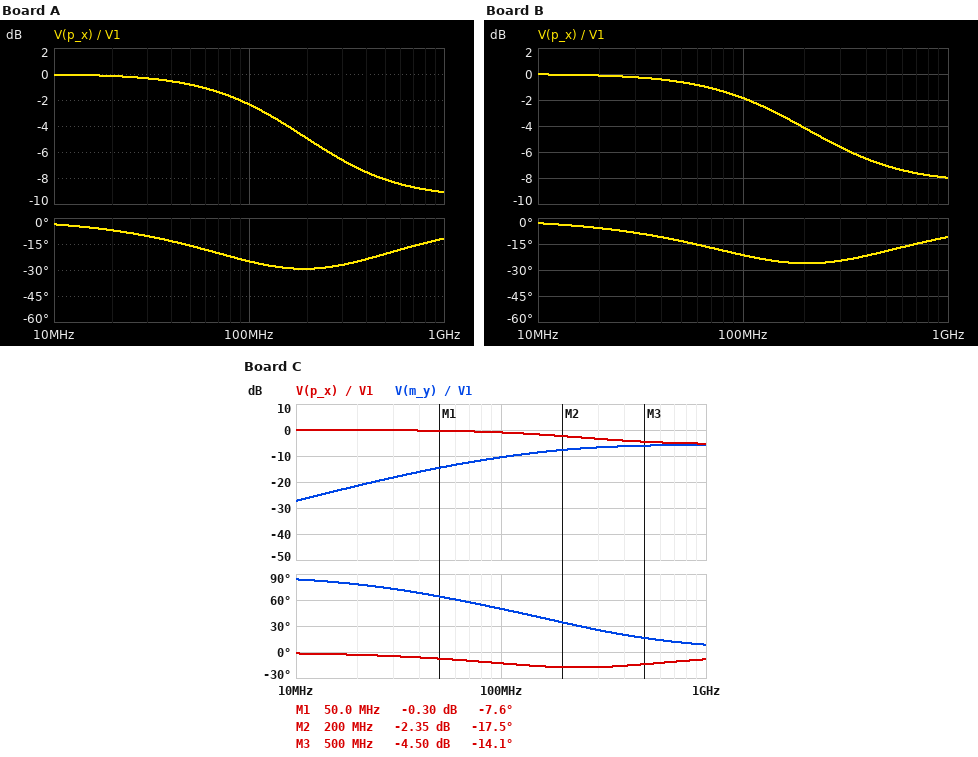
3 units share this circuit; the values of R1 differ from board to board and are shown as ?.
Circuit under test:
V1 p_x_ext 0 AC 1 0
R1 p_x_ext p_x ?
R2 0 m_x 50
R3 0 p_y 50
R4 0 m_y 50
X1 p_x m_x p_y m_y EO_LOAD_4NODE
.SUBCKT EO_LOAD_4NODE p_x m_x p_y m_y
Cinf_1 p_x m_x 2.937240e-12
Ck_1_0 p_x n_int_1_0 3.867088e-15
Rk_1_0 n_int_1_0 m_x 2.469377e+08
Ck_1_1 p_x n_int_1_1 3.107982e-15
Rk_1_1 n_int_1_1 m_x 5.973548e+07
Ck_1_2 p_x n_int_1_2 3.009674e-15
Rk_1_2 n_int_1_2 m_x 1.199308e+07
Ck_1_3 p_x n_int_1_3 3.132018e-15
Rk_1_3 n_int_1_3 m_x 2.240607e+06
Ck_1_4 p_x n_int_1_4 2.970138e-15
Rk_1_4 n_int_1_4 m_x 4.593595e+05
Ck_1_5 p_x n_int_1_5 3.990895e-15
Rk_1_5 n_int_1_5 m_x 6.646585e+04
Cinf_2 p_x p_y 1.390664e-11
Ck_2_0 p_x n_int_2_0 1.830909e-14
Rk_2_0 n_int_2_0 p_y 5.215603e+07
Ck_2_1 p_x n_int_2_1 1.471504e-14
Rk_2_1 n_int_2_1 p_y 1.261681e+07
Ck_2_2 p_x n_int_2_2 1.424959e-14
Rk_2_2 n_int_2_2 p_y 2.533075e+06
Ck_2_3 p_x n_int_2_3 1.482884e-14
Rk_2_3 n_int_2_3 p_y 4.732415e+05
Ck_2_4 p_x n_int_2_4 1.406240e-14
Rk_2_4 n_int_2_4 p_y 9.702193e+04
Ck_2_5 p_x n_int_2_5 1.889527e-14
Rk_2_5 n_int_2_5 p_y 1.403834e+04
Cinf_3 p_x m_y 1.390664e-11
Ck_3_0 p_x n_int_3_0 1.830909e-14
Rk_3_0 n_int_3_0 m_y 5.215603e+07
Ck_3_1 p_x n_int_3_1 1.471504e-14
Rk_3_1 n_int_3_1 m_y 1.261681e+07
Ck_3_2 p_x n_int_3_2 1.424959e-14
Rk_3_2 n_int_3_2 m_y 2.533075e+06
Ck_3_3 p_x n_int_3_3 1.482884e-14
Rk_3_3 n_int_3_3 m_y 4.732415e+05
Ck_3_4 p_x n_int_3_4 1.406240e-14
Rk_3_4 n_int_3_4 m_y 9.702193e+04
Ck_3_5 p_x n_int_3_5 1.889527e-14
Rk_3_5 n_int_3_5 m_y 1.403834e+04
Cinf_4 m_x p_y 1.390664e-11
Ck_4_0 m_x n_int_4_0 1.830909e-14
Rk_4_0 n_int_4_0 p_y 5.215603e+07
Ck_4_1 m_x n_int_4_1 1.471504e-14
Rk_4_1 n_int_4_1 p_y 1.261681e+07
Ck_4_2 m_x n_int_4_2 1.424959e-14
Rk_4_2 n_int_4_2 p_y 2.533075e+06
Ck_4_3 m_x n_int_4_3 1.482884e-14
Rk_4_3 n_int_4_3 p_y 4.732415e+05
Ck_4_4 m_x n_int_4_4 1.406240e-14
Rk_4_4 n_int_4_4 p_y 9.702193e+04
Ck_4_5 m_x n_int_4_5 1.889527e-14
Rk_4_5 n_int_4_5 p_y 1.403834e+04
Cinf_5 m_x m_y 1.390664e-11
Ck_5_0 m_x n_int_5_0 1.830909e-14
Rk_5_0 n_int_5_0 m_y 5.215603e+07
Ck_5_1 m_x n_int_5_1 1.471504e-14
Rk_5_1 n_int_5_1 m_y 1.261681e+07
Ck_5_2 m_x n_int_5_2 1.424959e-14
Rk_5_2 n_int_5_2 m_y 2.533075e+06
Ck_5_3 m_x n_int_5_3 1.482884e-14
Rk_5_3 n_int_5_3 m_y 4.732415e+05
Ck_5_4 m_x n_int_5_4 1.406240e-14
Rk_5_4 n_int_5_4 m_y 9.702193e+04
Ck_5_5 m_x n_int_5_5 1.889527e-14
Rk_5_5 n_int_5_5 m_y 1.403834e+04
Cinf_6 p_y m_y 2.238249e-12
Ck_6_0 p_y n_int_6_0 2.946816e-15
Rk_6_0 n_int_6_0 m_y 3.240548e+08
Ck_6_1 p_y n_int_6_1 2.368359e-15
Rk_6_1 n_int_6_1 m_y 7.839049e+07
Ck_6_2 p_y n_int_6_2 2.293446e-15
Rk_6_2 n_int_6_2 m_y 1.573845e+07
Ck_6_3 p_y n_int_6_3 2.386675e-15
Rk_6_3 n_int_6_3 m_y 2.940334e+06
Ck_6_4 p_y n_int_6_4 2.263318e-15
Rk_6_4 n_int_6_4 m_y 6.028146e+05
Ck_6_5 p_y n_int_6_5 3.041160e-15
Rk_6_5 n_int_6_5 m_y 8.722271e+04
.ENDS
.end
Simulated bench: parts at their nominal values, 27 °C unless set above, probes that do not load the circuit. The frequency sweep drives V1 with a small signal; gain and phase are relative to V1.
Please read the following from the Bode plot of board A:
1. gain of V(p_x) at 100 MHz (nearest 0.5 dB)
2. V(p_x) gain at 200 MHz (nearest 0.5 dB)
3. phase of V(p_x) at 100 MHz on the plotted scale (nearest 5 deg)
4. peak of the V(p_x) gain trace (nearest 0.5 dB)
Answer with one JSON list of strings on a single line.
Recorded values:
["-2.5 dB", "-5.0 dB", "-25 deg", "0 dB"]
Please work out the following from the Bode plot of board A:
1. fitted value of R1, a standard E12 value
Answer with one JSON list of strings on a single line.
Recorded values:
["33 Ω"]
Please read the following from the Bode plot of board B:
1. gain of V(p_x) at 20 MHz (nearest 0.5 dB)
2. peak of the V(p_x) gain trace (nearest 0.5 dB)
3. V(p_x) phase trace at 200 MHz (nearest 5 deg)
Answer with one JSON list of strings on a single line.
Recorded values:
["0 dB", "0 dB", "-25 deg"]
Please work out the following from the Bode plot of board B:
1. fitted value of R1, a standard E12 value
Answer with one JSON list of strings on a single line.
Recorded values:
["27 Ω"]
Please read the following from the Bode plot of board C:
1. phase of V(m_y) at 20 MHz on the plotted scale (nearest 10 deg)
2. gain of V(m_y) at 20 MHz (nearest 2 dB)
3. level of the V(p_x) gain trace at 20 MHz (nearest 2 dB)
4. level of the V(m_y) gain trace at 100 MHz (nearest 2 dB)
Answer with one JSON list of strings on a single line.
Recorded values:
["80 deg", "-22 dB", "0 dB", "-10 dB"]
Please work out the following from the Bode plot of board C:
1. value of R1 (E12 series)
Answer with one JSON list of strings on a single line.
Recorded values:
["15 Ω"]
